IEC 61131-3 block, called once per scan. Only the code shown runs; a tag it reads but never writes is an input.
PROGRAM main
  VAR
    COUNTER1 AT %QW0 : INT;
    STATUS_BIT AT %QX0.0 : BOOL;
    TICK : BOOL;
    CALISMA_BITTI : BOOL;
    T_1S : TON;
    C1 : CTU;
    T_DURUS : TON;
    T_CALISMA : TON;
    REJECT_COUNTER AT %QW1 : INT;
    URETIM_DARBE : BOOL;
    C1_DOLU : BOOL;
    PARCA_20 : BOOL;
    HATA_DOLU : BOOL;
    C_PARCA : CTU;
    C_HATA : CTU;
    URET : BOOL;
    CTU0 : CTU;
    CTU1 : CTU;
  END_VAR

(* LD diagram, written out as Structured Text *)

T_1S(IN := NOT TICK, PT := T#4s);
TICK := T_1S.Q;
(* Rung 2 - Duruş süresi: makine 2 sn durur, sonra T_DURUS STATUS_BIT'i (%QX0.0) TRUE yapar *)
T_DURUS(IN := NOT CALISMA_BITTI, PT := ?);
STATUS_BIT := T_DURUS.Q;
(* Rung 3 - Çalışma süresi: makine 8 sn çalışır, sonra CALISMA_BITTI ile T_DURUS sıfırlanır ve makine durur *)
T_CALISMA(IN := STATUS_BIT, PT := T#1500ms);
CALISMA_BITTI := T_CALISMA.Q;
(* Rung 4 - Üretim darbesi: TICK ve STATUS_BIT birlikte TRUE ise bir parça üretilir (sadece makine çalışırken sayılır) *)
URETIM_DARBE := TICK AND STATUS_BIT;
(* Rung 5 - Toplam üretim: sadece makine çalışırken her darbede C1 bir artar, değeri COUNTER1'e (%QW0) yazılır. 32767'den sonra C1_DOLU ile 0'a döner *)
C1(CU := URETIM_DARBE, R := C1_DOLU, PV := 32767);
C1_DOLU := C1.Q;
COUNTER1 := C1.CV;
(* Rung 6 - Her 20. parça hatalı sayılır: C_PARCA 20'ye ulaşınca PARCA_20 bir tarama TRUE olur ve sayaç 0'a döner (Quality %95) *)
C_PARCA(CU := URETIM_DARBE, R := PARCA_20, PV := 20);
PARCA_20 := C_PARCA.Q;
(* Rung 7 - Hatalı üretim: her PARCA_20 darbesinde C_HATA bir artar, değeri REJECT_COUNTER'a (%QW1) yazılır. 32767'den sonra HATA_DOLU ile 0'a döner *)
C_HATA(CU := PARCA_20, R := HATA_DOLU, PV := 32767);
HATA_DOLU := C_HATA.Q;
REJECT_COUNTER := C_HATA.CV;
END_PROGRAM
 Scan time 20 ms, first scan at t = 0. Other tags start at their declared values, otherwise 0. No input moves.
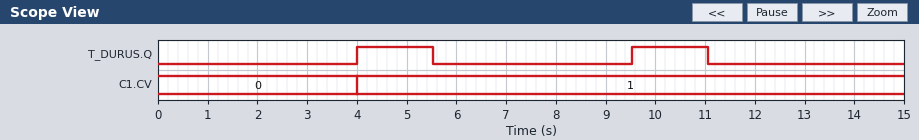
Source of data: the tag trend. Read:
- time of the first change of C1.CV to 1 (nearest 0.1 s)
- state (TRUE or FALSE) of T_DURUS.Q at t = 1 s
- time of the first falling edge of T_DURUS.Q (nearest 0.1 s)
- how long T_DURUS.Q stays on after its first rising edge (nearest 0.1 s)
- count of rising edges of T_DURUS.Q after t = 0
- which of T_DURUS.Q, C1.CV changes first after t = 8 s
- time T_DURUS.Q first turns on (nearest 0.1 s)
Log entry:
4.0 s
FALSE
5.5 s
1.5 s
2
T_DURUS.Q
4.0 s
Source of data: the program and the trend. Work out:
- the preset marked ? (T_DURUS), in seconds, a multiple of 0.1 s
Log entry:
4.0 s
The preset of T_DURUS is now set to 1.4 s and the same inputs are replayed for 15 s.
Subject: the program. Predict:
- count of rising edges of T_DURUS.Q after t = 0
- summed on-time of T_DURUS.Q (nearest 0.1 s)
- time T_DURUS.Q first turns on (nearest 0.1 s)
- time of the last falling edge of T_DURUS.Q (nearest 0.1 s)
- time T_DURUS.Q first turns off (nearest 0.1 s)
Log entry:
5
7.6 s
1.4 s
14.7 s
2.9 s
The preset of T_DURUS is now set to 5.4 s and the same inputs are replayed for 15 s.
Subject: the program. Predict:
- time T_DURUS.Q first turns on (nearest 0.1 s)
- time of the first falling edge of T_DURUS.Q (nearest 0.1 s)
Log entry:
5.4 s
6.9 s
